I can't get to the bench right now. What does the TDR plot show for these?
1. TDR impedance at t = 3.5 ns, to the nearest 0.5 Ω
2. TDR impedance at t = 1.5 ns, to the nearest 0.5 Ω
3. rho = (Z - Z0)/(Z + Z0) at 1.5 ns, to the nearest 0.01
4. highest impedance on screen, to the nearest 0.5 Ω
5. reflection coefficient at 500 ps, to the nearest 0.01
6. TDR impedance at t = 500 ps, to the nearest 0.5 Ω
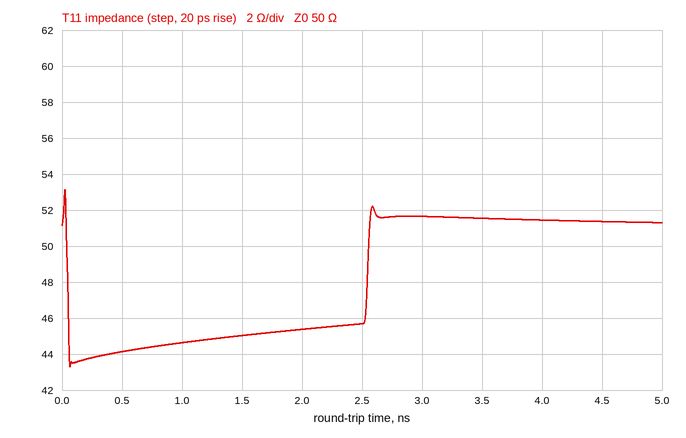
51.5 Ω
45.0 Ω
-0.05
53.0 Ω
-0.06
44.0 Ω
